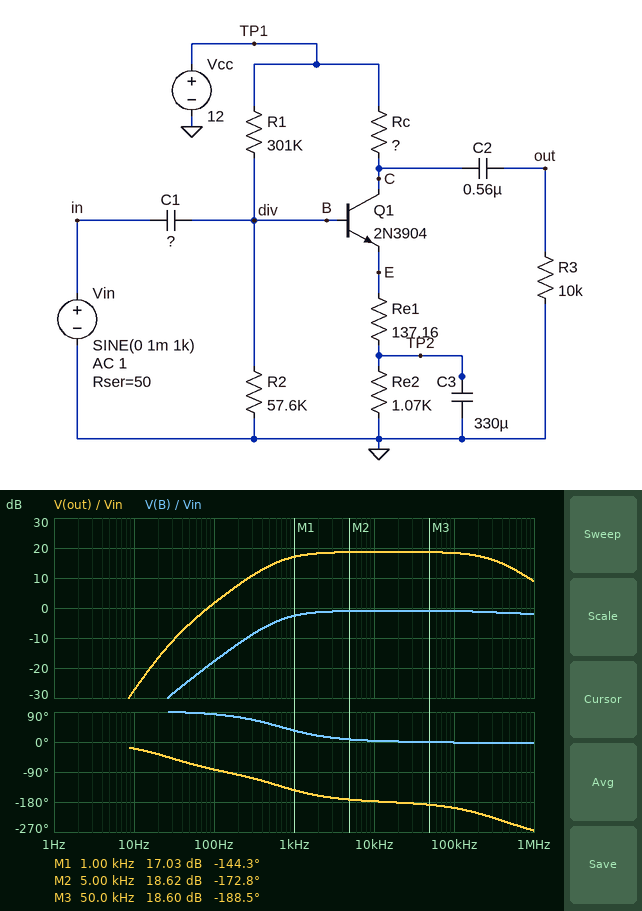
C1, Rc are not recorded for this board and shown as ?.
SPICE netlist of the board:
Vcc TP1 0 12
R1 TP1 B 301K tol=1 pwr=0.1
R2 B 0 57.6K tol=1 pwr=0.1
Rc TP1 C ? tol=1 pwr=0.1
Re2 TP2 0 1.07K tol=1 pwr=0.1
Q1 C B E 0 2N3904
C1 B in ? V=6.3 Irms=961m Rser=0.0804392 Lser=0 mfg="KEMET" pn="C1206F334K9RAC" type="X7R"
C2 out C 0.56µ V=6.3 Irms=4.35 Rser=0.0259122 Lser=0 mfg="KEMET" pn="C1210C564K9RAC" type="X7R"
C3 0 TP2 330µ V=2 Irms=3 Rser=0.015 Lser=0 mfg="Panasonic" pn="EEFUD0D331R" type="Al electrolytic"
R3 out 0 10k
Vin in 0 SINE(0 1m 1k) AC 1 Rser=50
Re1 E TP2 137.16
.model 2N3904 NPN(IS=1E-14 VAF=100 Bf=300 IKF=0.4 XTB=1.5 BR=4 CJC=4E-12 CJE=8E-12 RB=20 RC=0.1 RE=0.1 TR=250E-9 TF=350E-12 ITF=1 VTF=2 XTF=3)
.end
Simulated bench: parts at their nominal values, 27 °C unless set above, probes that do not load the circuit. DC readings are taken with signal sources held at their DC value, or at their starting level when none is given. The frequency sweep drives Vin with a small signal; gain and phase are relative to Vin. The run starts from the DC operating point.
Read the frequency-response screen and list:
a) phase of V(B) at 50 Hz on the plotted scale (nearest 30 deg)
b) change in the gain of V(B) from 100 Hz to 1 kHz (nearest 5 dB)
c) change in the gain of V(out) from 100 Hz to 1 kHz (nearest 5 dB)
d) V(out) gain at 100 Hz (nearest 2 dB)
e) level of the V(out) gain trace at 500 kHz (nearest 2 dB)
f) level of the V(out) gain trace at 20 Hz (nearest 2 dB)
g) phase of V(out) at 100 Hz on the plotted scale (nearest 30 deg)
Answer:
90 deg
15 dB
15 dB
2 dB
14 dB
-16 dB
-90 deg
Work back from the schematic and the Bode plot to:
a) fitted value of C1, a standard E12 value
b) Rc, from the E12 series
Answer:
470 nF
15 kΩ
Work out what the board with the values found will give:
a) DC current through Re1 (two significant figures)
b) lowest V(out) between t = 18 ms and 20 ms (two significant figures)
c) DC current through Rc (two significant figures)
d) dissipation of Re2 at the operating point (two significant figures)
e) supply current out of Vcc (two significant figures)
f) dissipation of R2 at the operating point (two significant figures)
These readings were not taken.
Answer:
740 µA
-6.8 mV
730 µA
590 µW
770 µA
41 µW
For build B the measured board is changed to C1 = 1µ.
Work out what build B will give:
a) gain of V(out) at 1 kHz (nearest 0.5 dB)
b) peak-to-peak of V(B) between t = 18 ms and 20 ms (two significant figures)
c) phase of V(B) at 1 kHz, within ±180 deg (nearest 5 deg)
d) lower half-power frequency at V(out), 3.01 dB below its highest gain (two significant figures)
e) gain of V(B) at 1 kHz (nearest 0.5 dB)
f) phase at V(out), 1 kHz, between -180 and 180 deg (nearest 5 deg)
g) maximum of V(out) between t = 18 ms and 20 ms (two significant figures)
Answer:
18.5 dB
1.7 mV
20 deg
320 Hz
-1.5 dB
-160 deg
9.0 mV
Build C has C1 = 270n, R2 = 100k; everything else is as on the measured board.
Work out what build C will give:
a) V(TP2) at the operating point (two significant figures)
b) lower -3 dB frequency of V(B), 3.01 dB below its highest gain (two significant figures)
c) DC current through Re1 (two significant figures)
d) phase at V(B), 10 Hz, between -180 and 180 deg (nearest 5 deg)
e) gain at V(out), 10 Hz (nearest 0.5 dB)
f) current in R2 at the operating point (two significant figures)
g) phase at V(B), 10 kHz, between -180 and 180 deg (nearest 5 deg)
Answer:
810 mV
1.5 kHz
750 µA
80 deg
-43.0 dB
16 µA
10 deg
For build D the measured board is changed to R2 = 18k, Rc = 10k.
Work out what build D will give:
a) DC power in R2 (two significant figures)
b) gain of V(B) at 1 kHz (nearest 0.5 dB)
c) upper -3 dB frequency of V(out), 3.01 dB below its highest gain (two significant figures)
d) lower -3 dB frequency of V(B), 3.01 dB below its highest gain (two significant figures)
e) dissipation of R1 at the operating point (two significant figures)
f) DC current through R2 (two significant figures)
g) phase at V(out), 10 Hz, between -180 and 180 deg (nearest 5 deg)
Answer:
25 µW
0 dB
16 MHz
22 Hz
430 µW
37 µA
-55 deg
